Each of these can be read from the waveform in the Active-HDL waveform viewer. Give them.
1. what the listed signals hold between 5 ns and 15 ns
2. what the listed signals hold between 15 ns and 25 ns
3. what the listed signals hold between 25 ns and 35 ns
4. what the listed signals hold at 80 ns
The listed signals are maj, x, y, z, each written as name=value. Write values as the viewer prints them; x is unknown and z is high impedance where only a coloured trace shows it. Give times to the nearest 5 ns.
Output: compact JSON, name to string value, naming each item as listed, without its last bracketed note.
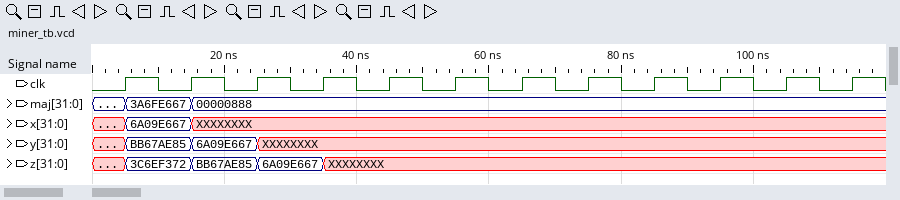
{"what the listed signals hold between 5 ns and 15 ns": "maj=3A6FE667, x=6A09E667, y=BB67AE85, z=3C6EF372", "what the listed signals hold between 15 ns and 25 ns": "maj=00000888, x=XXXXXXXX, y=6A09E667, z=BB67AE85", "what the listed signals hold between 25 ns and 35 ns": "maj=00000888, x=XXXXXXXX, y=XXXXXXXX, z=6A09E667", "what the listed signals hold at 80 ns": "maj=00000888, x=XXXXXXXX, y=XXXXXXXX, z=XXXXXXXX"}
